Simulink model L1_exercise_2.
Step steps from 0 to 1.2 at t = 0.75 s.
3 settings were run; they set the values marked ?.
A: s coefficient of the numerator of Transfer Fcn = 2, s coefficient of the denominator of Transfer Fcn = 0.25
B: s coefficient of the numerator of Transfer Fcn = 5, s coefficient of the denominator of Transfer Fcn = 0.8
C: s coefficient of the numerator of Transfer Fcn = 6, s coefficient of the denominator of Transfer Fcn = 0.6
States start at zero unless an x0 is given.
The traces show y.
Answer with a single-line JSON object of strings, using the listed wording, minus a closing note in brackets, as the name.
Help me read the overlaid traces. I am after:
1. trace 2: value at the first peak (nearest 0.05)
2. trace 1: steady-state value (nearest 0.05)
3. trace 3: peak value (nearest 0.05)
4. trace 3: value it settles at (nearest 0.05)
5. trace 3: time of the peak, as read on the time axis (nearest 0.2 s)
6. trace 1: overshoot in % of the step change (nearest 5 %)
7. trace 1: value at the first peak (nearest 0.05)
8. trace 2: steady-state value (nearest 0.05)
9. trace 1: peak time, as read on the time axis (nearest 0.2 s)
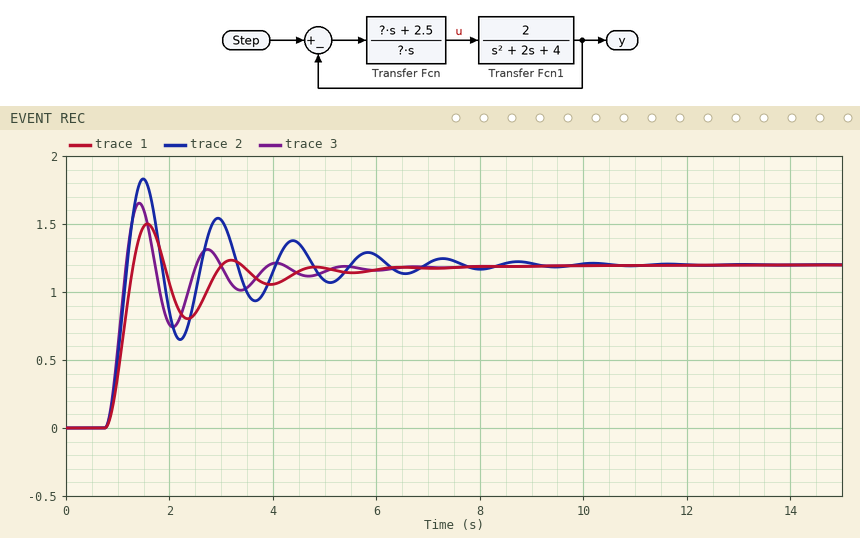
{"trace 2: value at the first peak": "1.85", "trace 1: steady-state value": "1.20", "trace 3: peak value": "1.65", "trace 3: value it settles at": "1.20", "trace 3: time of the peak, as read on the time axis": "1.4 s", "trace 1: overshoot in % of the step change": "25 %", "trace 1: value at the first peak": "1.50", "trace 2: steady-state value": "1.20", "trace 1: peak time, as read on the time axis": "1.6 s"}
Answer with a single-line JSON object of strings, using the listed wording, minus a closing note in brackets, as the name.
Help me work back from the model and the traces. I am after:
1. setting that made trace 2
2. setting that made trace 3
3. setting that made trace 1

{"setting that made trace 2": "A", "setting that made trace 3": "C", "setting that made trace 1": "B"}
